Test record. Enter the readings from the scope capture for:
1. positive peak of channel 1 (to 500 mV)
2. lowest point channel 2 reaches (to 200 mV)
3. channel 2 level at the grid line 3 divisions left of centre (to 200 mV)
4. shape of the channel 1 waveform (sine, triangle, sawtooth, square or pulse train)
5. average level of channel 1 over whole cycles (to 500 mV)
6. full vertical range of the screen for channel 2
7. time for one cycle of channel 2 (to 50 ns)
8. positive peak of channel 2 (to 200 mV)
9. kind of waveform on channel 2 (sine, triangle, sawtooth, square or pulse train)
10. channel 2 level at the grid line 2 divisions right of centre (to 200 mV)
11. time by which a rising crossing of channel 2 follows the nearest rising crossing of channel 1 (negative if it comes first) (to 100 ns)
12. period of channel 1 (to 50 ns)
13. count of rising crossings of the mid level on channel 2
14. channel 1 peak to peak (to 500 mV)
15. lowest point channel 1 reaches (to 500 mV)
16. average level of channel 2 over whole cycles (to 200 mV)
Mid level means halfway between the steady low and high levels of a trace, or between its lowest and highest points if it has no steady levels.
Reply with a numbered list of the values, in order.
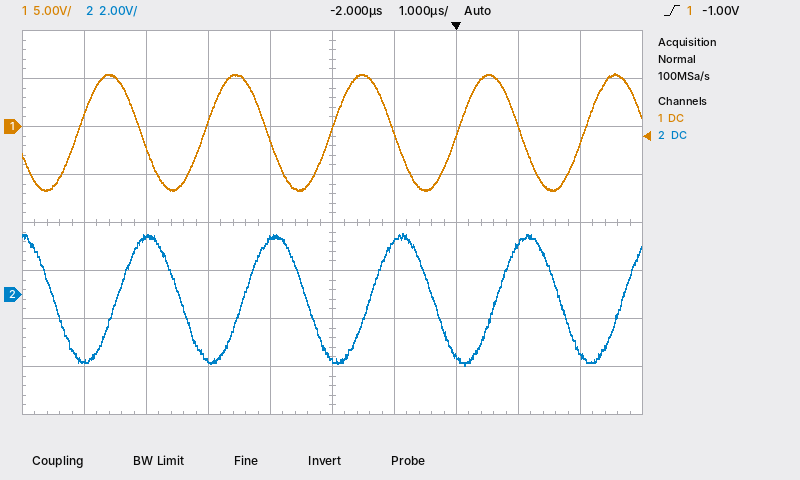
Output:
1. 5.5 V
2. -3.0 V
3. 2.4 V
4. sine
5. -500 mV
6. 16 V
7. 2.05 µs
8. 2.6 V
9. sine
10. -2.6 V
11. +600 ns
12. 2.05 µs
13. 5
14. 12.0 V
15. -6.5 V
16. -200 mV
